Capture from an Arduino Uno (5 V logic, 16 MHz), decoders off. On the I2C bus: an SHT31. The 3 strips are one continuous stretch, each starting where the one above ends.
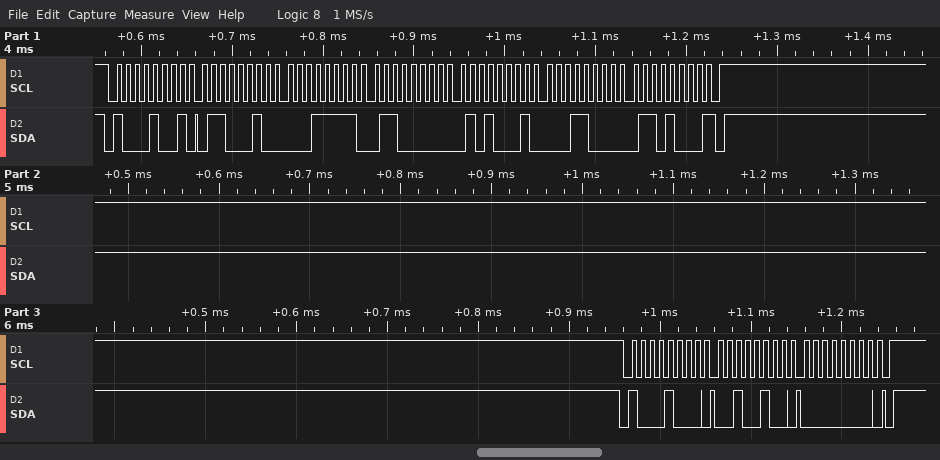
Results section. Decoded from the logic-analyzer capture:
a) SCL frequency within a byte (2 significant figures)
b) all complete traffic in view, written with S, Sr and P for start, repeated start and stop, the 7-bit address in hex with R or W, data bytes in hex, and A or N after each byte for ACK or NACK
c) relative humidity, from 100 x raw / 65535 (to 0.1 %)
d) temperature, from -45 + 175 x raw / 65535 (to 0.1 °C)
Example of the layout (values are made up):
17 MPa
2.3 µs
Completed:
100 kHz
S 44R A 62 A 1F A 60 A 51 A 18 A 68 N P S 44W A 24 A 00 A P
31.7 %
22.1 °C
